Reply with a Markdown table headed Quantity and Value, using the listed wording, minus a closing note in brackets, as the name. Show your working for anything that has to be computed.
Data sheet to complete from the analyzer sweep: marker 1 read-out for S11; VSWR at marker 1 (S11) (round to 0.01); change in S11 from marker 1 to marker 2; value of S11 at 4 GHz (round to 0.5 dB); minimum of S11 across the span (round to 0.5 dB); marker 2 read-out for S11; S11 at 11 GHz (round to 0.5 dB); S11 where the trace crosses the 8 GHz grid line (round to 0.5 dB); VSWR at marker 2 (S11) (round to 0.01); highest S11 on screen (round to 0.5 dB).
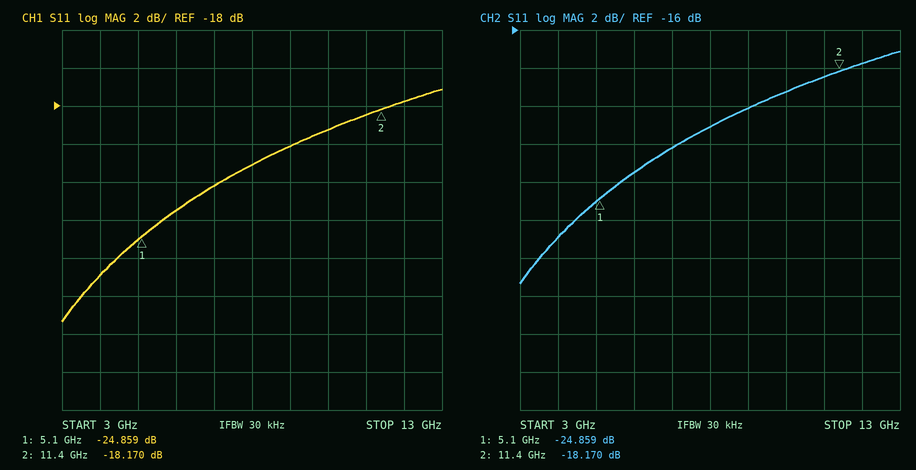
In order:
| Quantity | Value |
|---|---|
| marker 1 read-out for S11 | -24.859 dB |
| VSWR at marker 1 (S11) | (1 + 0.0572)/(1 − 0.0572) ≈ 1.12 |
| change in S11 from marker 1 to marker 2 | -18.17 − (-24.859) = 6.689 dB |
| value of S11 at 4 GHz | -27.0 dB |
| minimum of S11 across the span | -29.5 dB |
| marker 2 read-out for S11 | -18.170 dB |
| S11 at 11 GHz | -18.5 dB |
| S11 where the trace crosses the 8 GHz grid line | -21.0 dB |
| VSWR at marker 2 (S11) | (1 + 0.1235)/(1 − 0.1235) ≈ 1.28 |
| highest S11 on screen | -17.0 dB |
